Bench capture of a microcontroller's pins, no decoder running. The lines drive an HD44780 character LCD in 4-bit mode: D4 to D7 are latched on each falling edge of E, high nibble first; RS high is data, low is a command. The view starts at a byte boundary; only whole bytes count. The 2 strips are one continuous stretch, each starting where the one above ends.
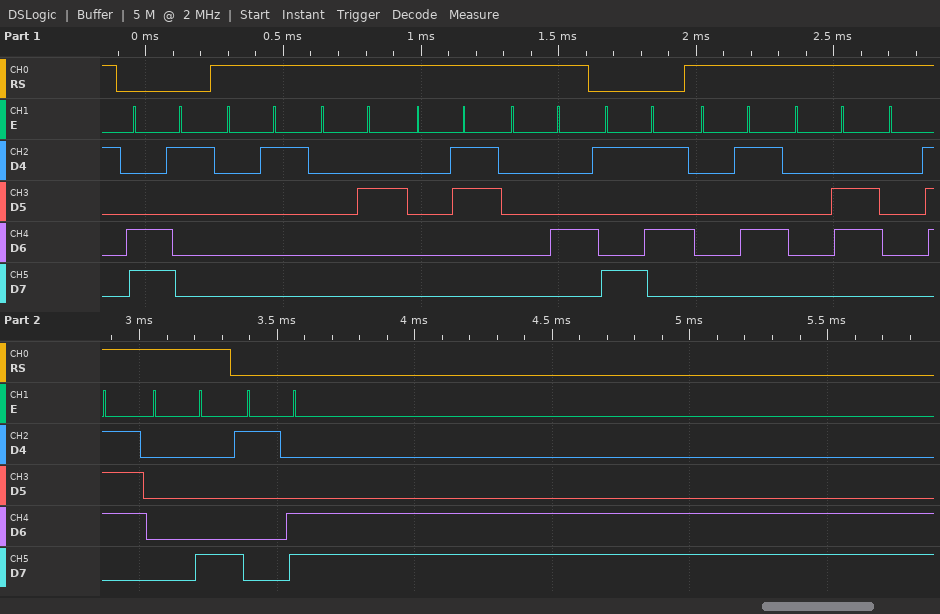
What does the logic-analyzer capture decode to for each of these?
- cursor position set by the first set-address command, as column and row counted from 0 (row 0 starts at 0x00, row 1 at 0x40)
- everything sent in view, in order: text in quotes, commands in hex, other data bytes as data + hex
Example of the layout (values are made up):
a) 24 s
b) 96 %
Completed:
a) column 1, row 1
b) 0xC1 data 01 02 03 04 0x95 data 05 06 07 08 0x1C
